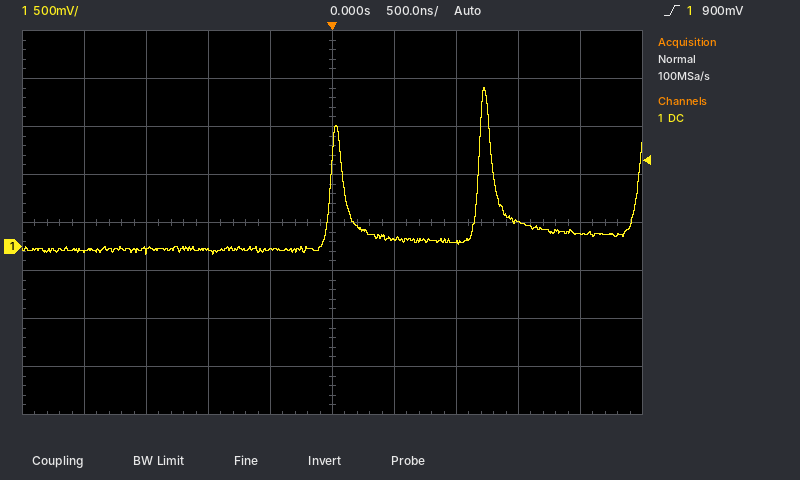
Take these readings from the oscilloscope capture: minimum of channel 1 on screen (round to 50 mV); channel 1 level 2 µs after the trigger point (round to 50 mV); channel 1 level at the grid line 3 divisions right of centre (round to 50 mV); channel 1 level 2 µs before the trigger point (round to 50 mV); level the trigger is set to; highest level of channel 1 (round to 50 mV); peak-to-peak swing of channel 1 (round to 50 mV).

-100 mV
150 mV
250 mV
-50 mV
900 mV
1.65 V
1.75 V
